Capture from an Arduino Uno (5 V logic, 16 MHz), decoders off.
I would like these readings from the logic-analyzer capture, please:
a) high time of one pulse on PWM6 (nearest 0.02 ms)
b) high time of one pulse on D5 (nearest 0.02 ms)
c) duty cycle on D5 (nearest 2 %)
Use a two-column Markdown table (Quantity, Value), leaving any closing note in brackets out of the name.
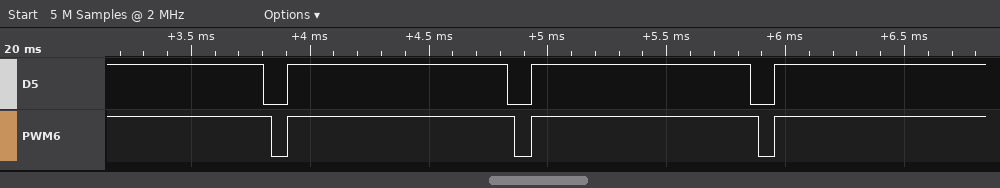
| Quantity | Value |
|---|---|
| high time of one pulse on PWM6 | 0.96 ms |
| high time of one pulse on D5 | 0.92 ms |
| duty cycle on D5 | 90 % |
